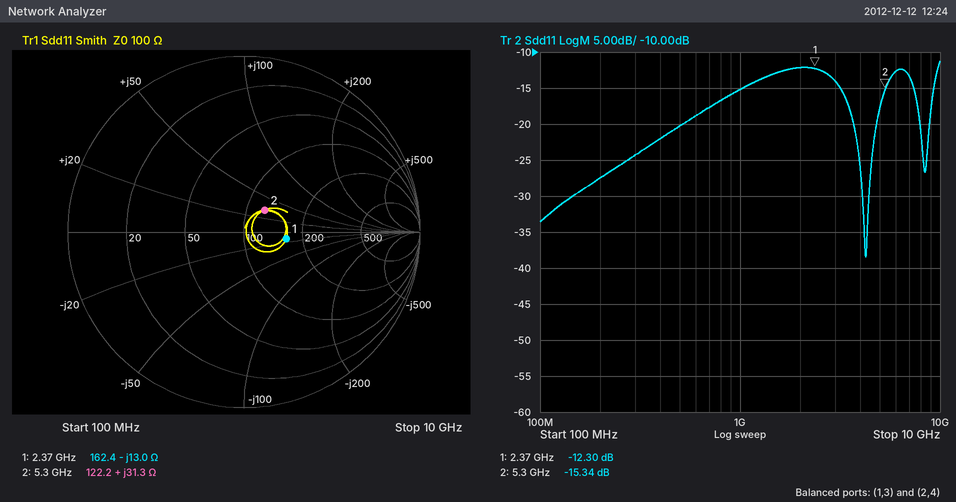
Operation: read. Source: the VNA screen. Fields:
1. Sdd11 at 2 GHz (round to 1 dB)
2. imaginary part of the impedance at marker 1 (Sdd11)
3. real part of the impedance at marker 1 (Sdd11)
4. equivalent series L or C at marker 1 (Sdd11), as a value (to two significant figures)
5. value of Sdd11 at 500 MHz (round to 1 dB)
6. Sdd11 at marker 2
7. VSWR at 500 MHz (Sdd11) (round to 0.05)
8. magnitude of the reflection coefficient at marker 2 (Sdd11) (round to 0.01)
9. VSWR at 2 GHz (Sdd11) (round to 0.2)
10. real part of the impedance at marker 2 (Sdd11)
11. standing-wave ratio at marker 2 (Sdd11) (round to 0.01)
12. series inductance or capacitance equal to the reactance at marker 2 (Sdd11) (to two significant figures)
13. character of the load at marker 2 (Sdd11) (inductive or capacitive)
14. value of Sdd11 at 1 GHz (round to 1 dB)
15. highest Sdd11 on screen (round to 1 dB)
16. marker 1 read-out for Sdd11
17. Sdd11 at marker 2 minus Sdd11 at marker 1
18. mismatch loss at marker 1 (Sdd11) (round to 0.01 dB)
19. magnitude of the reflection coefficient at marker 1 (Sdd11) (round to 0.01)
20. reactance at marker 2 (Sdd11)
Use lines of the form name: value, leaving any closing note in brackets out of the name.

Sdd11 at 2 GHz: -12 dB
imaginary part of the impedance at marker 1: -13.0 Ω
real part of the impedance at marker 1: 162.4 Ω
equivalent series L or C at marker 1 (Sdd11), as a value: 5.2 pF
value of Sdd11 at 500 MHz: -20 dB
Sdd11 at marker 2: -15.34 dB
VSWR at 500 MHz (Sdd11): 1.20
magnitude of the reflection coefficient at marker 2 (Sdd11): 0.17
VSWR at 2 GHz (Sdd11): 1.6
real part of the impedance at marker 2: 122.2 Ω
standing-wave ratio at marker 2 (Sdd11): 1.41
series inductance or capacitance equal to the reactance at marker 2 (Sdd11): 940 pH
character of the load at marker 2 (Sdd11): inductive
value of Sdd11 at 1 GHz: -15 dB
highest Sdd11 on screen: -11 dB
marker 1 read-out for Sdd11: -12.30 dB
Sdd11 at marker 2 minus Sdd11 at marker 1: -3.04 dB
mismatch loss at marker 1 (Sdd11): 0.26 dB
magnitude of the reflection coefficient at marker 1 (Sdd11): 0.24
reactance at marker 2: +31.3 Ω
